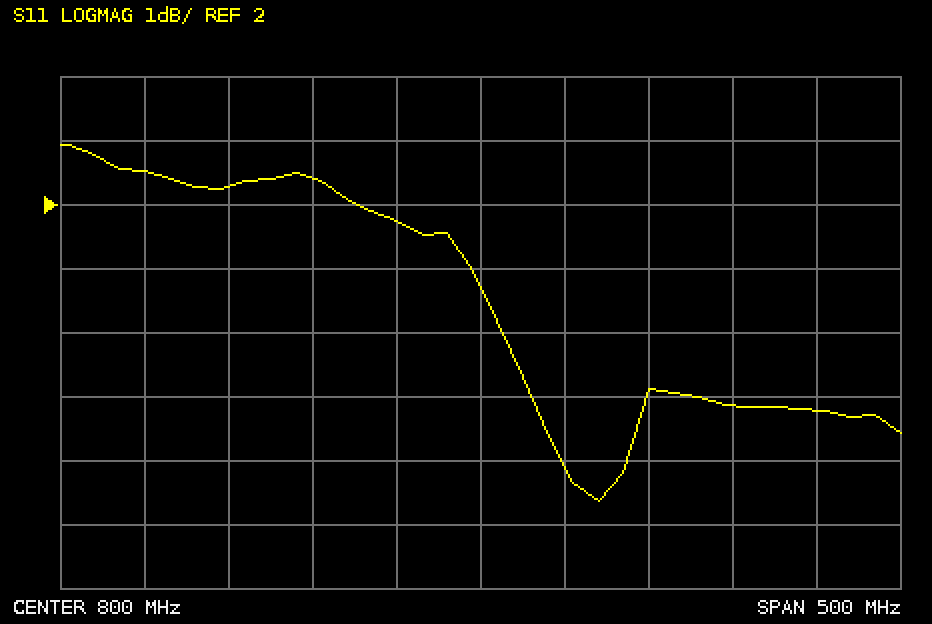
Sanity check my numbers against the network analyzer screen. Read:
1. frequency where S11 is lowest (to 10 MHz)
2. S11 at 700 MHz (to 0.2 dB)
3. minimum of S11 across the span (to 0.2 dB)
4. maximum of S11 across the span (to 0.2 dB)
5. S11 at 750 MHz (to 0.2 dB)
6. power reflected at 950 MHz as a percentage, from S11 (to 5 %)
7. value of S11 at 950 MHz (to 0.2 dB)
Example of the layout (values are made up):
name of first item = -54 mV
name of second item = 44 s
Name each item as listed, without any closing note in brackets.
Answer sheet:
frequency where S11 is lowest = 870 MHz
S11 at 700 MHz = 2.4 dB
minimum of S11 across the span = -2.6 dB
maximum of S11 across the span = 3.0 dB
S11 at 750 MHz = 1.8 dB
power reflected at 950 MHz as a percentage, from S11 = 75 %
value of S11 at 950 MHz = -1.2 dB
